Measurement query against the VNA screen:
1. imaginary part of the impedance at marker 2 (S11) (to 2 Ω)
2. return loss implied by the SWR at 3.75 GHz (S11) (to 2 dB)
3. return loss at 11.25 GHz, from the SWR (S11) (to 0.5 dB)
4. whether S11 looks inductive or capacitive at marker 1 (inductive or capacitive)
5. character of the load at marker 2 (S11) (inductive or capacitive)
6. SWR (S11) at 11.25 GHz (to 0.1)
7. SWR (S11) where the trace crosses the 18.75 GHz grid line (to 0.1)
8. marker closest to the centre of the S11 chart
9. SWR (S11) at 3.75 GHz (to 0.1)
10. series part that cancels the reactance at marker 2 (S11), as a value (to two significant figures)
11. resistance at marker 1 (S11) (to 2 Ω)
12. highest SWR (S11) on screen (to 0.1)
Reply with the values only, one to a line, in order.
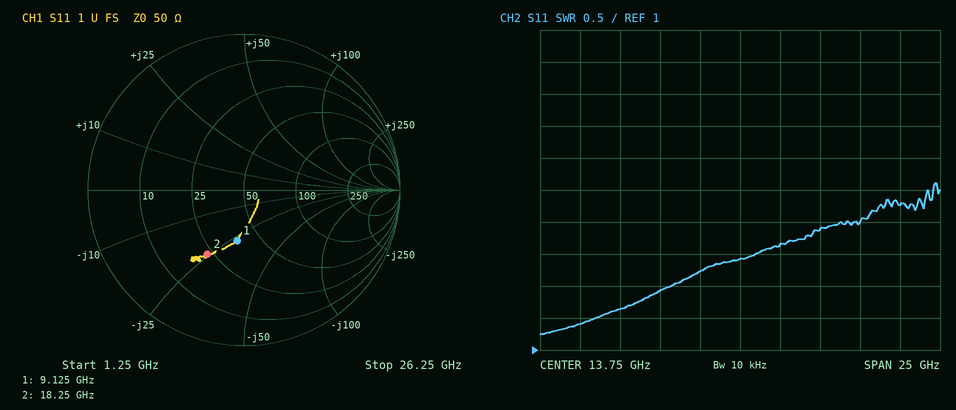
-24 Ω
16 dB
8.5 dB
capacitive
capacitive
2.2
2.9
marker 1
1.4
210 pH
38 Ω
3.6
